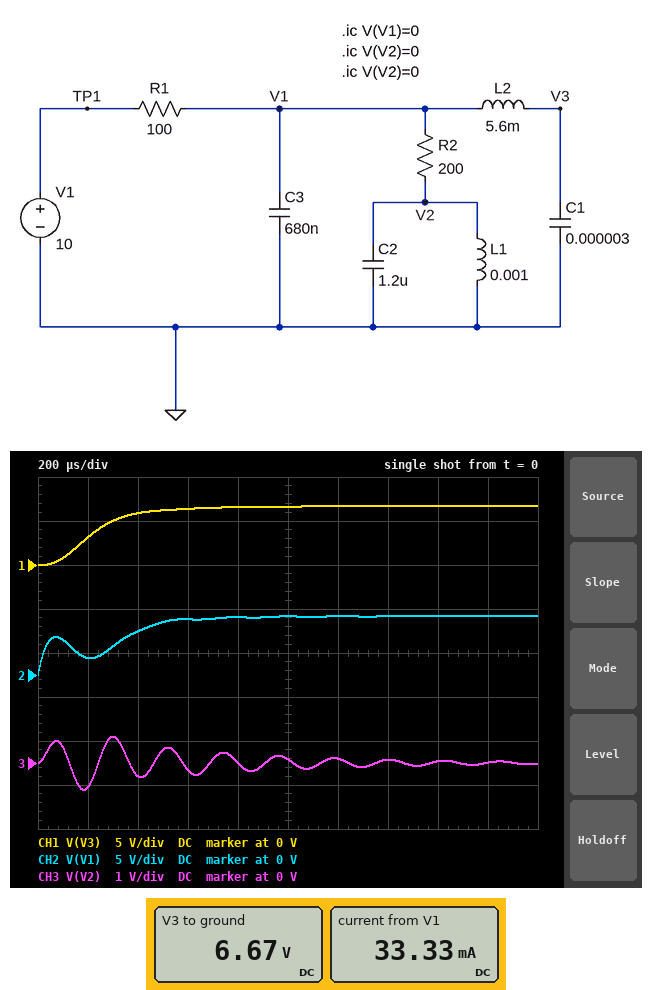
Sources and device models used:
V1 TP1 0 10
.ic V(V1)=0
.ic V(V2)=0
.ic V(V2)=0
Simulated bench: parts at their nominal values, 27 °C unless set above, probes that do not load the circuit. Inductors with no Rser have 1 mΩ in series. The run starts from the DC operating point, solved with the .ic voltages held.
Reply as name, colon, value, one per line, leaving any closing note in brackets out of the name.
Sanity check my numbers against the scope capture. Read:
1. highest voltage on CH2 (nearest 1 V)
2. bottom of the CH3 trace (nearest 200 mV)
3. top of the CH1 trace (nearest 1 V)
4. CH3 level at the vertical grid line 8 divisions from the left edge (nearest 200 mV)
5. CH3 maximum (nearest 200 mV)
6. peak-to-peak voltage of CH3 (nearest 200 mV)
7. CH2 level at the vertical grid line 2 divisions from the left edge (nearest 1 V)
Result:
highest voltage on CH2: 7 V
bottom of the CH3 trace: -600 mV
top of the CH1 trace: 7 V
CH3 level at the vertical grid line 8 divisions from the left edge: 0 V
CH3 maximum: 600 mV
peak-to-peak voltage of CH3: 1.2 V
CH2 level at the vertical grid line 2 divisions from the left edge: 5 V
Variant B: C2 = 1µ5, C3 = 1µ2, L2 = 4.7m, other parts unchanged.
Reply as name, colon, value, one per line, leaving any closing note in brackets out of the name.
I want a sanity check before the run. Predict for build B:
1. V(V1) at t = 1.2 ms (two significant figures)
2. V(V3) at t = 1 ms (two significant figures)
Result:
V(V1) at t = 1.2 ms: 6.6 V
V(V3) at t = 1 ms: 6.5 V
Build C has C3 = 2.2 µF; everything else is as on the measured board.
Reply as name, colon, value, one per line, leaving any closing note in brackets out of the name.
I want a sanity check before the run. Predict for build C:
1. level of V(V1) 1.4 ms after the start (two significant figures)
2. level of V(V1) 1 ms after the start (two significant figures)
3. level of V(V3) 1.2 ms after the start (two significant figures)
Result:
level of V(V1) 1.4 ms after the start: 6.5 V
level of V(V1) 1 ms after the start: 6.1 V
level of V(V3) 1.2 ms after the start: 6.4 V
